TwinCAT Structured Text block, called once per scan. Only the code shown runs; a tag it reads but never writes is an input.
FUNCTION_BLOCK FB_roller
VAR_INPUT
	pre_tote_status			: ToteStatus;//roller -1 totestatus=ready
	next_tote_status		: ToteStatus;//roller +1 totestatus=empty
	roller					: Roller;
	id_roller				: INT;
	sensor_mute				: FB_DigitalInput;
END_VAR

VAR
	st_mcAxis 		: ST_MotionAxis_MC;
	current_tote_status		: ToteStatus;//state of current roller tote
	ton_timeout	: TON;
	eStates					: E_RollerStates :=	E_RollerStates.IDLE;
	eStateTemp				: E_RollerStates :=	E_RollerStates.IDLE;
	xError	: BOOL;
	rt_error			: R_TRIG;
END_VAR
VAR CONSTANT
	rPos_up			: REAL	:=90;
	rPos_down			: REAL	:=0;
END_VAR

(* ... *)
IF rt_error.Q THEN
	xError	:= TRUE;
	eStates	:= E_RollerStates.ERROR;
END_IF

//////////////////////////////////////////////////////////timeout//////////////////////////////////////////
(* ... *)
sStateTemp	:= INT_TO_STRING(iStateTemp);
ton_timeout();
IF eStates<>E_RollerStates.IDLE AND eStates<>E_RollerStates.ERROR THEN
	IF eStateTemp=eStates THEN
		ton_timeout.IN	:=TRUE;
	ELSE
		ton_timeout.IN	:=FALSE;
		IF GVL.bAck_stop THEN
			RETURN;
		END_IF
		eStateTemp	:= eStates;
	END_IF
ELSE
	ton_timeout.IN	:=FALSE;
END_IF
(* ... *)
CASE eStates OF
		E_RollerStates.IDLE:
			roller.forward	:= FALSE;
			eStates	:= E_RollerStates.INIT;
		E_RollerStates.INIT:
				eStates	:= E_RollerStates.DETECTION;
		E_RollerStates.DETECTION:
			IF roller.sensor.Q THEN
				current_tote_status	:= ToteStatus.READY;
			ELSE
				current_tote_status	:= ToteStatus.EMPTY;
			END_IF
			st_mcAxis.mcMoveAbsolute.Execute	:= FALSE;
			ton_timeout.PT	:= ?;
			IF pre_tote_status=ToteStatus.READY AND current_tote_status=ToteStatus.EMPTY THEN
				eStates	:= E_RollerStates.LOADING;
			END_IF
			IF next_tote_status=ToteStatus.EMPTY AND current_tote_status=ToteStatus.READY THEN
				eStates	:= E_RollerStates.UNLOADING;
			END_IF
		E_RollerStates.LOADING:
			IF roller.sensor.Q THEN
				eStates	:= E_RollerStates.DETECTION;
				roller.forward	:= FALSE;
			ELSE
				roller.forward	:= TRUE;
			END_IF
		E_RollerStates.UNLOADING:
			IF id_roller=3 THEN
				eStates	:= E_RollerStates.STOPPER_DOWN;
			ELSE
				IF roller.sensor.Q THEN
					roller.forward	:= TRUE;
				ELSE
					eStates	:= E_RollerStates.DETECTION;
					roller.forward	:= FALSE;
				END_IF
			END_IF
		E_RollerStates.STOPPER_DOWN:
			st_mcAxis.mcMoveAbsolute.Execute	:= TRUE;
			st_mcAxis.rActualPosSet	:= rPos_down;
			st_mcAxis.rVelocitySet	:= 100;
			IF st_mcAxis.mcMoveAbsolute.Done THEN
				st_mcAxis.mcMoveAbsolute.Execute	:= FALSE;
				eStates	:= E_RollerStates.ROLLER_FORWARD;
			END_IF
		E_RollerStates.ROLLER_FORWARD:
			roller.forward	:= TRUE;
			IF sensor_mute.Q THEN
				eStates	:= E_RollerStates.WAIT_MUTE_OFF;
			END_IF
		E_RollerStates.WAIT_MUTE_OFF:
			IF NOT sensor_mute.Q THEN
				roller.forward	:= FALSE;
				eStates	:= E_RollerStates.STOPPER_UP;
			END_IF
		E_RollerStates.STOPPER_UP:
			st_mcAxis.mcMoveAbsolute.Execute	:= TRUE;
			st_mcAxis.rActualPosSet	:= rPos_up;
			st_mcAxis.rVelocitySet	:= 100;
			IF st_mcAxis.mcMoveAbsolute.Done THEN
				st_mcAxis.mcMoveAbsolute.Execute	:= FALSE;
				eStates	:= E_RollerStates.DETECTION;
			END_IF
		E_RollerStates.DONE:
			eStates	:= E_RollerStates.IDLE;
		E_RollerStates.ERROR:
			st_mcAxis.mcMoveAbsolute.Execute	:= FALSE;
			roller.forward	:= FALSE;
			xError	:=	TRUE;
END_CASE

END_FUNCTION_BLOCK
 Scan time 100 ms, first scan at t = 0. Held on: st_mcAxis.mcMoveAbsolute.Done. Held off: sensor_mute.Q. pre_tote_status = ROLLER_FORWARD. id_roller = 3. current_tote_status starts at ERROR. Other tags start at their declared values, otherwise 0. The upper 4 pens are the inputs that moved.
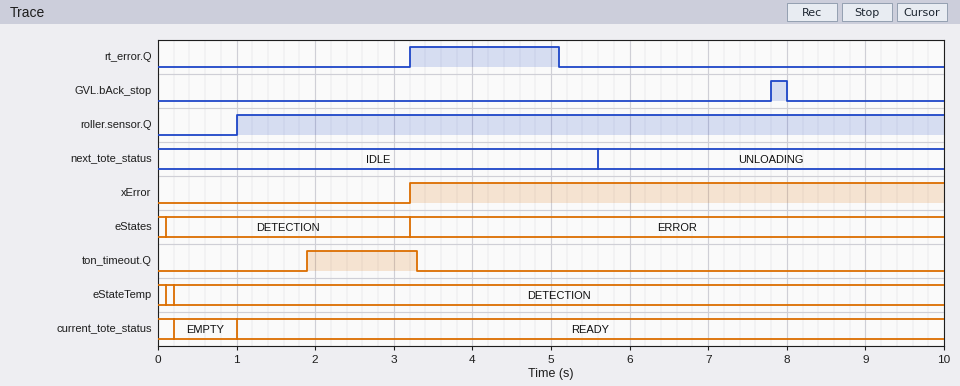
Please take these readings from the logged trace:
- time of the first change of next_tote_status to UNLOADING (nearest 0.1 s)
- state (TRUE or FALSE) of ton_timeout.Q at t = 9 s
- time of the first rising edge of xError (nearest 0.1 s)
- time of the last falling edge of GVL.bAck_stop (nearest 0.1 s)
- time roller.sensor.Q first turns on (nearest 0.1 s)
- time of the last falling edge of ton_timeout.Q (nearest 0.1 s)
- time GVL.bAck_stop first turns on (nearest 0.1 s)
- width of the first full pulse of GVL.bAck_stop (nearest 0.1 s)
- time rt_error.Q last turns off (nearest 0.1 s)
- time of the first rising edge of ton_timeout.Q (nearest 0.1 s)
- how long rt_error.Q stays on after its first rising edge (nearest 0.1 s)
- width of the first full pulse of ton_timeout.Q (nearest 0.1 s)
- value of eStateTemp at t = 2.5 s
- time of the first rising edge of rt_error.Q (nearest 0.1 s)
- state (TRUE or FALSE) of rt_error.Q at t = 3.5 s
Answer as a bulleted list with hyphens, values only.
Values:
- 5.6 s
- FALSE
- 3.2 s
- 8.0 s
- 1.0 s
- 3.3 s
- 7.8 s
- 0.2 s
- 5.1 s
- 1.9 s
- 1.9 s
- 1.4 s
- DETECTION
- 3.2 s
- TRUE
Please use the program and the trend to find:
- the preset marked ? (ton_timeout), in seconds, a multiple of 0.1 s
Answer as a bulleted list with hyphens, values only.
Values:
- 1.5 s
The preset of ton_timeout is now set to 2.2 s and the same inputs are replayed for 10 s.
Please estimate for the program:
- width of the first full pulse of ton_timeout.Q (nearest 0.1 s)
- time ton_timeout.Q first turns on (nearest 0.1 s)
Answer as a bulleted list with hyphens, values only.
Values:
- 0.7 s
- 2.6 s
